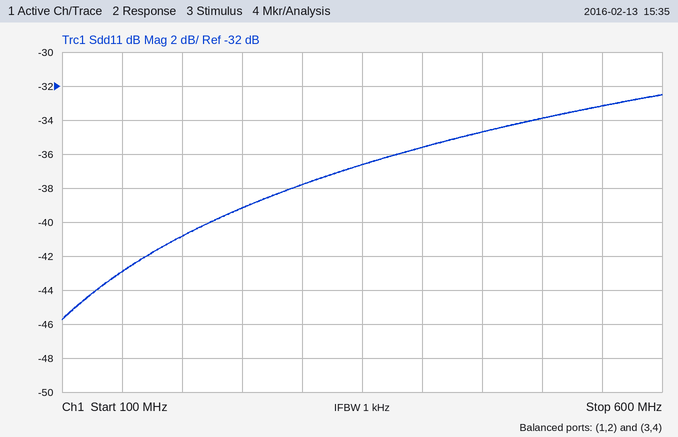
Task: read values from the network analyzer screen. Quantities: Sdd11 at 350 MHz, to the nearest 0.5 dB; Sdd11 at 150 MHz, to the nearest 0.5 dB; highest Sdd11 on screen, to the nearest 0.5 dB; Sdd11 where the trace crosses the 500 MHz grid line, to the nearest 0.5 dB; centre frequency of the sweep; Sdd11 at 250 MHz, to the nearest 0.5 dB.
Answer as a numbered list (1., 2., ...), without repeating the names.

1. -36.5 dB
2. -43.0 dB
3. -32.5 dB
4. -34.0 dB
5. 350 MHz
6. -39.0 dB
